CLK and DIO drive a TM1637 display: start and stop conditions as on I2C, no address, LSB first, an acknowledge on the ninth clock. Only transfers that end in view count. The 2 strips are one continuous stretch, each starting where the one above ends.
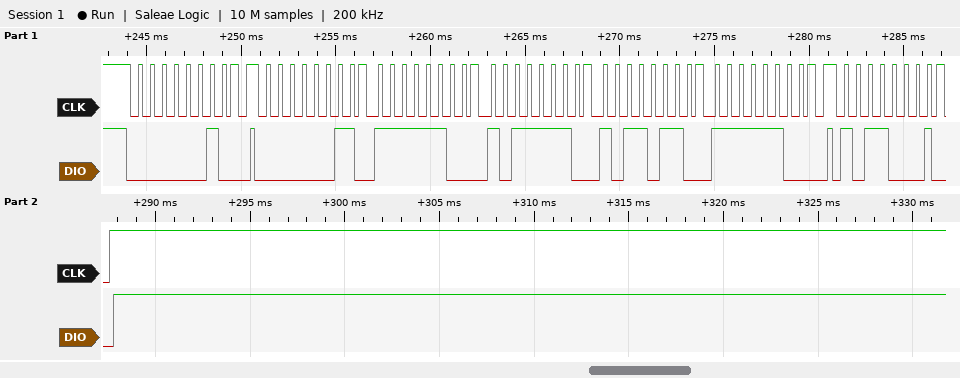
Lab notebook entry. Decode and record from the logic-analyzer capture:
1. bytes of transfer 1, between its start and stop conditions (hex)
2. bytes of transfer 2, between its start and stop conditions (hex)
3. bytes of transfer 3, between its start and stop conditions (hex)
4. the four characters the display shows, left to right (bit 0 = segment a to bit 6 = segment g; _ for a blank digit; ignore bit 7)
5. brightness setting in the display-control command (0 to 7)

40
C0 3F 7D 6D 3F
8D
0650
5
